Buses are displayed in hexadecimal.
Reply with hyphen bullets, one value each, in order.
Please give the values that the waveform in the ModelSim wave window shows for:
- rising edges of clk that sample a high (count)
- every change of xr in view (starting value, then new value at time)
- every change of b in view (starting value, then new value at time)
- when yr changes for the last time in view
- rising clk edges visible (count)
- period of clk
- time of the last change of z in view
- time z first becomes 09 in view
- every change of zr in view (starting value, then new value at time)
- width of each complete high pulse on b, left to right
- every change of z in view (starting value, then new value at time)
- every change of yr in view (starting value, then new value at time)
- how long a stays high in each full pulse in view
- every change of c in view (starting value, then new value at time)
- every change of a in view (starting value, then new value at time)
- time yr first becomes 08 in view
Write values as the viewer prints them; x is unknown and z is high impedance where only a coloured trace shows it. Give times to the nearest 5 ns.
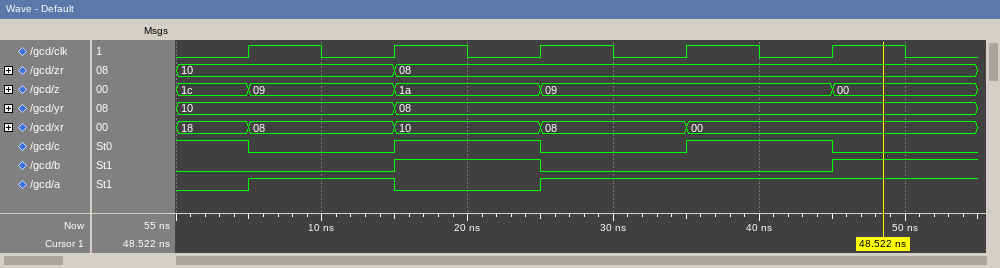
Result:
- 3
- 18, 08 at 5 ns, 10 at 15 ns, 08 at 25 ns, 00 at 35 ns
- 0, 1 at 15 ns, 0 at 25 ns, 1 at 45 ns
- 15 ns
- 5
- 10 ns
- 45 ns
- 5 ns
- 10, 08 at 15 ns
- 10 ns
- 1c, 09 at 5 ns, 1a at 15 ns, 09 at 25 ns, 00 at 45 ns
- 10, 08 at 15 ns
- 10 ns
- 1, 0 at 5 ns, 1 at 15 ns, 0 at 25 ns, 1 at 35 ns, 0 at 45 ns
- 0, 1 at 5 ns, 0 at 15 ns, 1 at 25 ns
- 15 ns
